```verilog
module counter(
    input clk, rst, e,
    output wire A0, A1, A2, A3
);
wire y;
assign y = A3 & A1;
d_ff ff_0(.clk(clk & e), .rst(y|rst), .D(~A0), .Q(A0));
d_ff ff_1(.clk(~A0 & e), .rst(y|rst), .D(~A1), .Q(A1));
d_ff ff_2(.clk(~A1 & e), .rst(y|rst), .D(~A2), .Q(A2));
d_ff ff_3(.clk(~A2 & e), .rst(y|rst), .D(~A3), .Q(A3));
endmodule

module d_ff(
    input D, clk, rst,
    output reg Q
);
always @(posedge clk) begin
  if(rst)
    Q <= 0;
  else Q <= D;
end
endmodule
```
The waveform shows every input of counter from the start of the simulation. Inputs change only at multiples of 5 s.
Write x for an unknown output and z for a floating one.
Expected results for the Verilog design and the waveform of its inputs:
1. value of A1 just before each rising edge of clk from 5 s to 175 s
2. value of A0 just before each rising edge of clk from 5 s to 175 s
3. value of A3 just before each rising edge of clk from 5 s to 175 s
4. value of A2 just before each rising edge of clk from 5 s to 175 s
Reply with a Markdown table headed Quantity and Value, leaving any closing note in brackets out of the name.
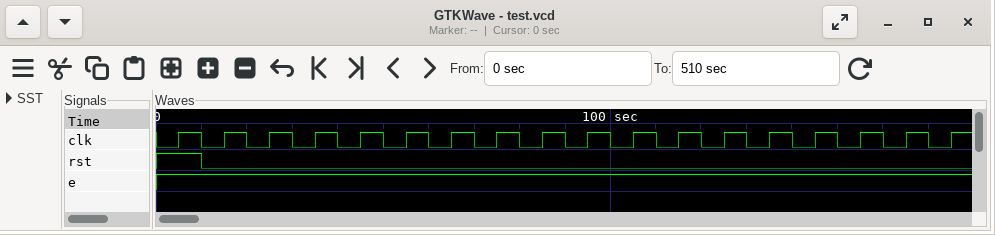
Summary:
| Quantity | Value |
|---|---|
| value of A1 just before each rising edge of clk from 5 s to 175 s | x 0 0 1 1 0 0 1 1 0 0 1 1 1 1 1 1 1 |
| value of A0 just before each rising edge of clk from 5 s to 175 s | x 0 1 0 1 0 1 0 1 0 1 0 0 0 0 0 0 0 |
| value of A3 just before each rising edge of clk from 5 s to 175 s | x 0 0 0 0 0 0 0 0 1 1 1 1 1 1 1 1 1 |
| value of A2 just before each rising edge of clk from 5 s to 175 s | x 0 0 0 0 1 1 1 1 0 0 0 0 0 0 0 0 0 |
